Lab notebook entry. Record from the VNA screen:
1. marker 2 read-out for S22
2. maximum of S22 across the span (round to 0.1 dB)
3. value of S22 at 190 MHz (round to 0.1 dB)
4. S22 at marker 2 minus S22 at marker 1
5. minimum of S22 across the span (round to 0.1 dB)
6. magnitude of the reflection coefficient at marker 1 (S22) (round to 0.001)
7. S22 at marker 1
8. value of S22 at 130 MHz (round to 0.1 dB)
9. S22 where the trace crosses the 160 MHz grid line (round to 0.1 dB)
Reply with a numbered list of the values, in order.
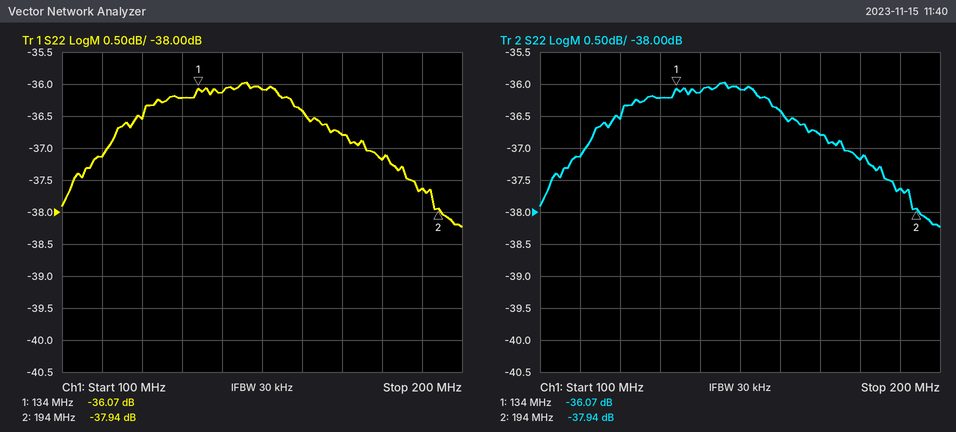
1. -37.94 dB
2. -36.0 dB
3. -37.6 dB
4. -1.87 dB
5. -38.2 dB
6. 0.016
7. -36.07 dB
8. -36.2 dB
9. -36.4 dB
